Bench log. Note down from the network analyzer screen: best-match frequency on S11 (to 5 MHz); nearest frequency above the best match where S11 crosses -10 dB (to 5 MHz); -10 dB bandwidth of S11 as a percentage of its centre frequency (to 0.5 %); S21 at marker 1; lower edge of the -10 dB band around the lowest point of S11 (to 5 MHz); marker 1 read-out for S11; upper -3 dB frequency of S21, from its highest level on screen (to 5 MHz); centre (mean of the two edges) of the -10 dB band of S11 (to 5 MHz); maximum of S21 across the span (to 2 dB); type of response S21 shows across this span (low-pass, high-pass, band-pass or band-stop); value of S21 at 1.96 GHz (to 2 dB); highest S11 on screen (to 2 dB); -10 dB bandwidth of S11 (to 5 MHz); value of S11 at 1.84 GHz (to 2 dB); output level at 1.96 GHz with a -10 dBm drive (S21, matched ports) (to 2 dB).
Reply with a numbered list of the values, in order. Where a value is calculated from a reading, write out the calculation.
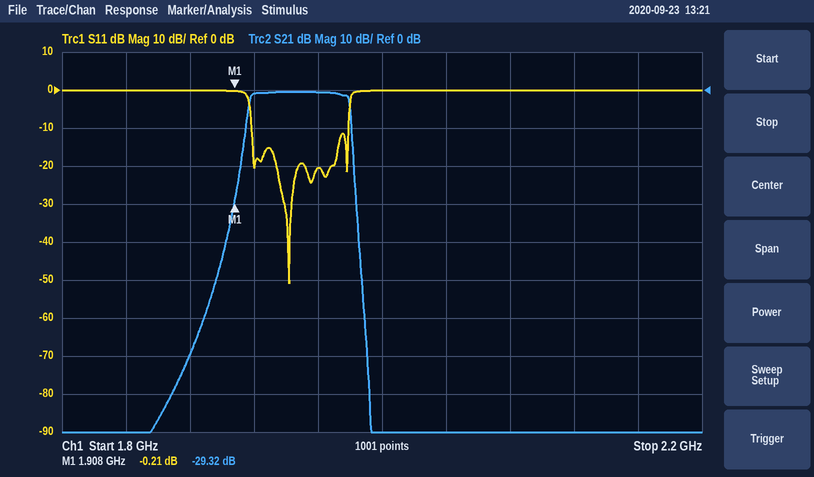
1. 1.940 GHz
2. 1.980 GHz
3. 60 MHz / 1.95 GHz ≈ 3.08 %, so 3.0 % to the nearest 0.5 %
4. -29.32 dB
5. 1.920 GHz
6. -0.21 dB
7. 1.980 GHz
8. 1.950 GHz
9. 0 dB
10. band-pass
11. 0 dB
12. 0 dB
13. 1.980 GHz − 1.920 GHz = 60 MHz
14. 0 dB
15. -10 dBm + (0 dB) = -10 dBm
